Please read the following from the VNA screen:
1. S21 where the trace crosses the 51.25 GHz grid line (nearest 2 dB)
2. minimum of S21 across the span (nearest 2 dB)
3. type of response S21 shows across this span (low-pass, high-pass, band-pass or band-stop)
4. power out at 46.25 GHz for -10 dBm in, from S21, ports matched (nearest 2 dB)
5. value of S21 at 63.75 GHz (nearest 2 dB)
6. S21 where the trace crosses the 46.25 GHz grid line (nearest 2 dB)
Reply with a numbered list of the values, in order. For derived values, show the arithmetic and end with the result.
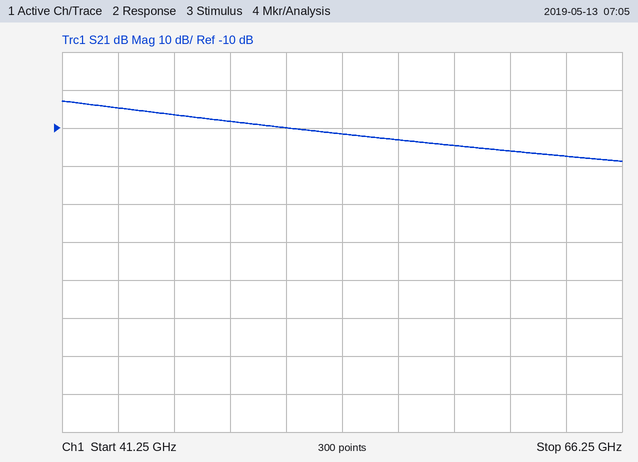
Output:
1. -10 dB
2. -18 dB
3. low-pass
4. -10 dBm + (-6 dB) = -16 dBm
5. -18 dB
6. -6 dB
